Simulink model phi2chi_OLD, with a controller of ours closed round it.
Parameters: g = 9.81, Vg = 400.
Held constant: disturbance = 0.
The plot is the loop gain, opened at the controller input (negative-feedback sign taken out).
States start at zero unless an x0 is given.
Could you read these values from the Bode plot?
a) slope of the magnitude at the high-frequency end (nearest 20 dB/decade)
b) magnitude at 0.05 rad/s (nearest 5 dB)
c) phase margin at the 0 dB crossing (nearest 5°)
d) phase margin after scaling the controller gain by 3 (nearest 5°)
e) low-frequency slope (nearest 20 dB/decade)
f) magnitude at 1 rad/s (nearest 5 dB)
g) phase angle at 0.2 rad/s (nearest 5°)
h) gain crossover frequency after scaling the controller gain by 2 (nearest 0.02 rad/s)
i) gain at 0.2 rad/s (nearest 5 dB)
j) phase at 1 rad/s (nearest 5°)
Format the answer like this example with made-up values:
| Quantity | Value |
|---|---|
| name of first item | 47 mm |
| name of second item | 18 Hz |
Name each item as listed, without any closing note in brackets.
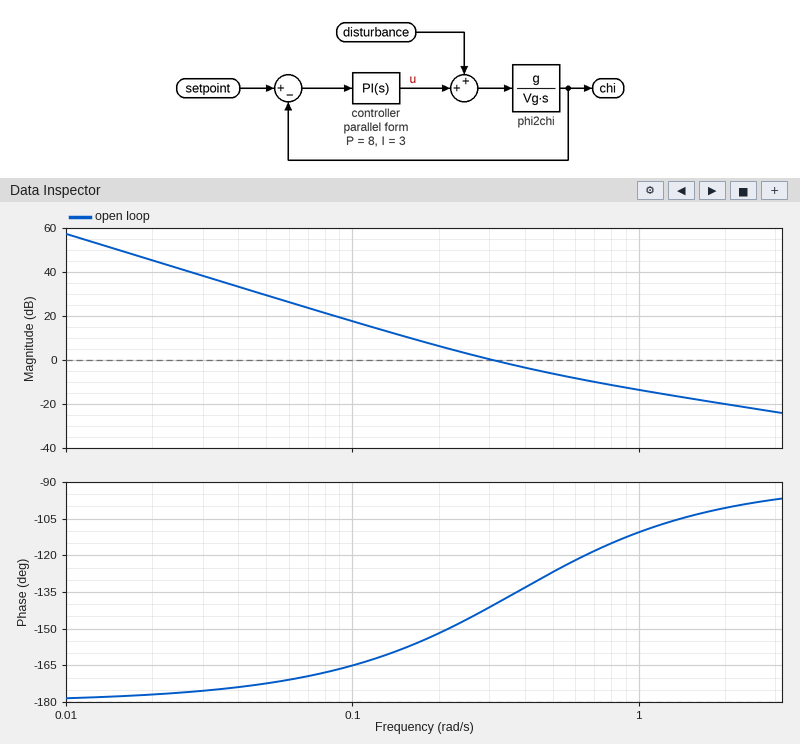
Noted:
| Quantity | Value |
|---|---|
| slope of the magnitude at the high-frequency end | -20 dB/decade |
| magnitude at 0.05 rad/s | 30 dB |
| phase margin at the 0 dB crossing | 40° |
| phase margin after scaling the controller gain by 3 | 60° |
| low-frequency slope | -40 dB/decade |
| magnitude at 1 rad/s | -15 dB |
| phase angle at 0.2 rad/s | -150° |
| gain crossover frequency after scaling the controller gain by 2 | 0.50 rad/s |
| gain at 0.2 rad/s | 5 dB |
| phase at 1 rad/s | -110° |
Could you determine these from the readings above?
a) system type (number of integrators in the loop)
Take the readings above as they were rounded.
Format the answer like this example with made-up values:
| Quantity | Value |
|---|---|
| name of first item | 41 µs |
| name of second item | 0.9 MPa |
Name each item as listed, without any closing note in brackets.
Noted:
| Quantity | Value |
|---|---|
| system type | 2 |
